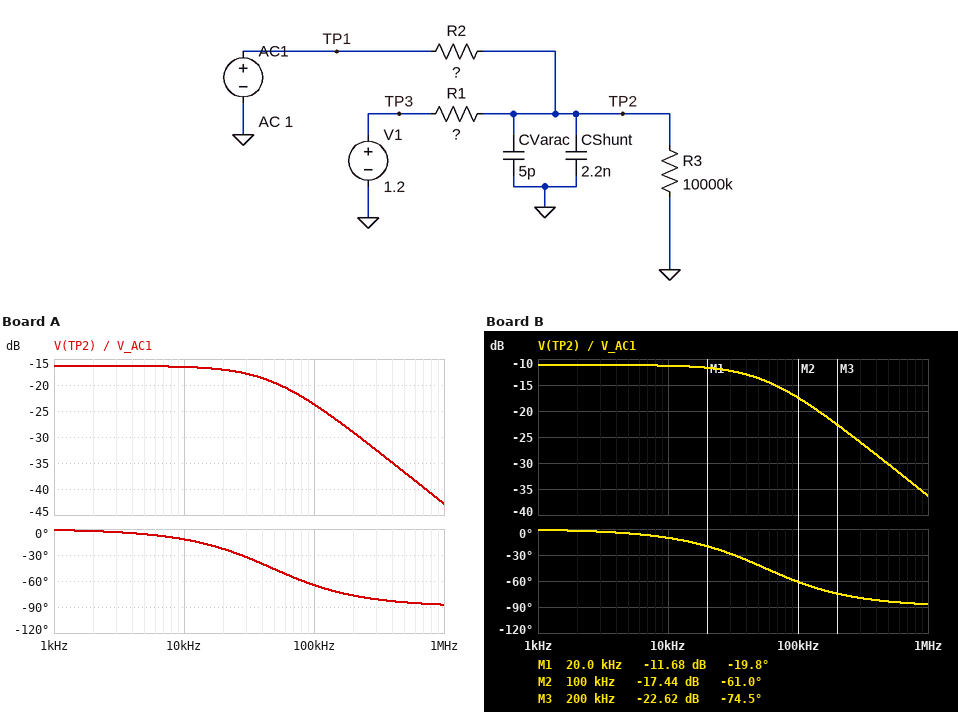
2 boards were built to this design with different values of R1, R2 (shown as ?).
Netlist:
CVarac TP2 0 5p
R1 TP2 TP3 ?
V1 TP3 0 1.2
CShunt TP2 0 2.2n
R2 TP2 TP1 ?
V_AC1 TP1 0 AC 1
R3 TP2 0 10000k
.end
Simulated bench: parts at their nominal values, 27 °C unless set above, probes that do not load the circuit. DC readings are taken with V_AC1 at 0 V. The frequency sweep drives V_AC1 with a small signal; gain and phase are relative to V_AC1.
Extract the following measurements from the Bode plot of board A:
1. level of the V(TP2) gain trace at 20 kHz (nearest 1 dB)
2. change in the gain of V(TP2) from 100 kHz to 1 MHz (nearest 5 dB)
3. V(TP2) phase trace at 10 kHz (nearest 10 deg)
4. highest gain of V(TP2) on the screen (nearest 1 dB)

-17 dB
-20 dB
-10 deg
-16 dB
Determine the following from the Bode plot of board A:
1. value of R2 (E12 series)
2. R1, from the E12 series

10 kΩ
1.8 kΩ
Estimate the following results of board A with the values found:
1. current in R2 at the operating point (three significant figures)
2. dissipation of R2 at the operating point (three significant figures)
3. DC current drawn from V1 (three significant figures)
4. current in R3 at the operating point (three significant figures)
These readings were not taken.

102 µA
103 µW
102 µA
102 nA
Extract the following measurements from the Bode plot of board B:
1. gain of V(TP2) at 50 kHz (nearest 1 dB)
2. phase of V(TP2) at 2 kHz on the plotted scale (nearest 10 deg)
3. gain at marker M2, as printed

-14 dB
0 deg
-17.44 dB
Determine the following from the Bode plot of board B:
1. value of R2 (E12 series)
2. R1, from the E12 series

4.7 kΩ
1.8 kΩ
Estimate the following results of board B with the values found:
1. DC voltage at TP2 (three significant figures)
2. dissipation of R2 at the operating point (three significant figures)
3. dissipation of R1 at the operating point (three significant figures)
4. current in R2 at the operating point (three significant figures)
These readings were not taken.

868 mV
160 µW
61.4 µW
185 µA
